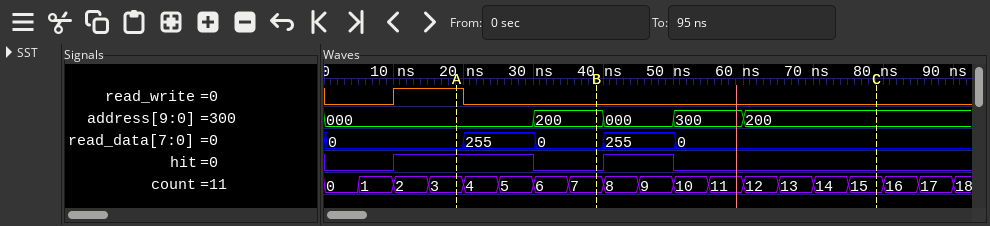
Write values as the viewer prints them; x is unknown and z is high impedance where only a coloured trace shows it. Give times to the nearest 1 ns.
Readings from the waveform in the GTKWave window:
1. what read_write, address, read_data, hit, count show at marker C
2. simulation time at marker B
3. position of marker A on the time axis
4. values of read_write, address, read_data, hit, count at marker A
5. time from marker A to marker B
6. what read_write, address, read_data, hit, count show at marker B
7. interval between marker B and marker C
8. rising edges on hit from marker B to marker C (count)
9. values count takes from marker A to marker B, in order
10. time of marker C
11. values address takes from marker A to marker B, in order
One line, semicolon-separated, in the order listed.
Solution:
read_write=0, address=200, read_data=0, hit=0, count=15; 39 ns; 19 ns; read_write=1, address=000, read_data=0, hit=1, count=3; 20 ns; read_write=0, address=200, read_data=0, hit=0, count=7; 40 ns; 1; 3, 4, 5, 6, 7; 79 ns; 000, 200
